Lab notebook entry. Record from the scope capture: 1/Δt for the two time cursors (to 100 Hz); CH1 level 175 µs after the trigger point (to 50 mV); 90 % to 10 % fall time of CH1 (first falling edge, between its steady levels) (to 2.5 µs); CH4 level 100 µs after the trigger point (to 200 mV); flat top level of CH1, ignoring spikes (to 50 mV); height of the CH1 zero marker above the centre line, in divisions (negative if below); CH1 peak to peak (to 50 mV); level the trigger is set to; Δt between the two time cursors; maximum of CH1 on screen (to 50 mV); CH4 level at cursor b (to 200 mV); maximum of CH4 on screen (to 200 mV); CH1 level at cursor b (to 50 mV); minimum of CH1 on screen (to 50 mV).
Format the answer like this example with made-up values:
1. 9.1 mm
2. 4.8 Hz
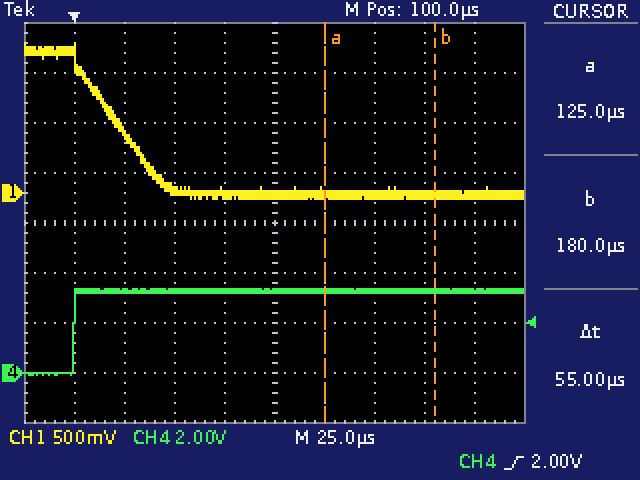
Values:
1. 18.2 kHz
2. 0 mV
3. 42.5 µs
4. 3.2 V
5. 1.40 V
6. +0.6 div
7. 1.55 V
8. 2.00 V
9. 55 µs
10. 1.50 V
11. 3.2 V
12. 3.4 V
13. 0 mV
14. -50 mV
